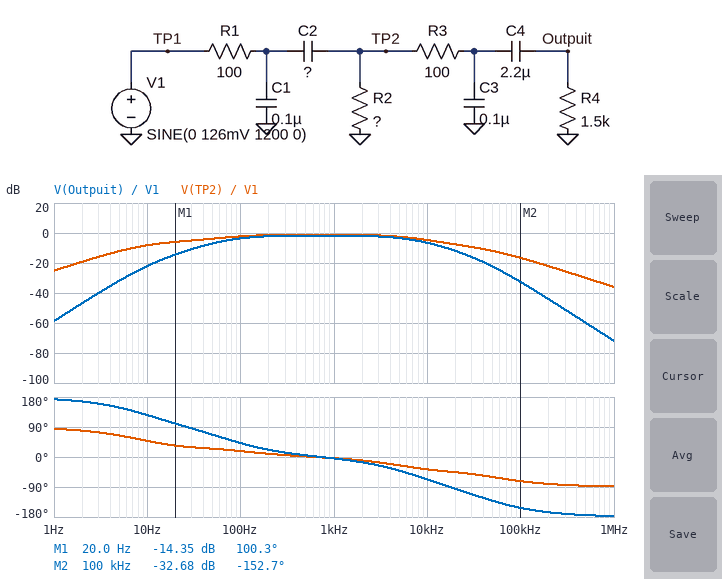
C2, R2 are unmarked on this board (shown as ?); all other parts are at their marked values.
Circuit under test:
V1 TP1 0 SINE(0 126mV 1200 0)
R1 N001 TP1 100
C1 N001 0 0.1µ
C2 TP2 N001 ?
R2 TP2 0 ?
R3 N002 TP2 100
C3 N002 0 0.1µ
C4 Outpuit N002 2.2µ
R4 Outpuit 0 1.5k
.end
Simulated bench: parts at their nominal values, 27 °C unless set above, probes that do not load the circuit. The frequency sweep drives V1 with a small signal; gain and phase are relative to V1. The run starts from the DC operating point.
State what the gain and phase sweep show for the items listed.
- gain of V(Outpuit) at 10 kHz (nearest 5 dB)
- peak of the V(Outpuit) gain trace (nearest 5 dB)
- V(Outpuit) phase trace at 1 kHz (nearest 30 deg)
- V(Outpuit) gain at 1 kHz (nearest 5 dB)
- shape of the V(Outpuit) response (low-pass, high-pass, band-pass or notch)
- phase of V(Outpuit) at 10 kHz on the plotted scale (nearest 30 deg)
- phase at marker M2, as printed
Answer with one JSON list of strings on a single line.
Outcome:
["-5 dB", "0 dB", "0 deg", "0 dB", "band-pass", "-60 deg", "-152.7 deg"]
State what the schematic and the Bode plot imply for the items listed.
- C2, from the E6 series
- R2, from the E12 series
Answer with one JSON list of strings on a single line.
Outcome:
["3.3 µF", "2.7 kΩ"]
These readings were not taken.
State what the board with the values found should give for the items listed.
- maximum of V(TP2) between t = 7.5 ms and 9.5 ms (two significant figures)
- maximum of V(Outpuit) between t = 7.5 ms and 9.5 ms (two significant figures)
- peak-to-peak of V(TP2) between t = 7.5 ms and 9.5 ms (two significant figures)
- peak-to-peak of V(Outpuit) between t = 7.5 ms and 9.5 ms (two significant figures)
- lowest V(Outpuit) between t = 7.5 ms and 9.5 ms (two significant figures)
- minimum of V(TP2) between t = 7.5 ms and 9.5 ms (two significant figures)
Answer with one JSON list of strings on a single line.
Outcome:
["110 mV", "100 mV", "220 mV", "210 mV", "-100 mV", "-110 mV"]
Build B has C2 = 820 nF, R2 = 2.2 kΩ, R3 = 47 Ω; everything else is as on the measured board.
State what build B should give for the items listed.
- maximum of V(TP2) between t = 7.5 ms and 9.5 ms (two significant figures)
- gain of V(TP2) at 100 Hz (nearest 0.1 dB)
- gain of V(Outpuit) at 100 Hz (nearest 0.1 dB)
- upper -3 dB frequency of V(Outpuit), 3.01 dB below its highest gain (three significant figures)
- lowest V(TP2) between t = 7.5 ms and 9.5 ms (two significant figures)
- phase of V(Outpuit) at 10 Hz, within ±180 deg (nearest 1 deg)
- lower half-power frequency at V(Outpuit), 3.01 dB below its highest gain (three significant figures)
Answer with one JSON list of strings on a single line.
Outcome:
["100 mV", "-8.1 dB", "-9.2 dB", "8.64 kHz", "-100 mV", "146 deg", "196 Hz"]
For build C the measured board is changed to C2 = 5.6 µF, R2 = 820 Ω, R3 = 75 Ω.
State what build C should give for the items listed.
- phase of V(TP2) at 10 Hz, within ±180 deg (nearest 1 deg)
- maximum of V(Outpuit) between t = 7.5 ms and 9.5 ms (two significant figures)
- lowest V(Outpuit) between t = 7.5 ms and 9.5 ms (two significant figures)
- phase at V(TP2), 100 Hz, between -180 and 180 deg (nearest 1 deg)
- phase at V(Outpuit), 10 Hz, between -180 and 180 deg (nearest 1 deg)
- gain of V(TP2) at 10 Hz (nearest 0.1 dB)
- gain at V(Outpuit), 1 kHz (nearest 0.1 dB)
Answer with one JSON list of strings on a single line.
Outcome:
["67 deg", "99 mV", "-99 mV", "20 deg", "144 deg", "-11.7 dB", "-2.1 dB"]
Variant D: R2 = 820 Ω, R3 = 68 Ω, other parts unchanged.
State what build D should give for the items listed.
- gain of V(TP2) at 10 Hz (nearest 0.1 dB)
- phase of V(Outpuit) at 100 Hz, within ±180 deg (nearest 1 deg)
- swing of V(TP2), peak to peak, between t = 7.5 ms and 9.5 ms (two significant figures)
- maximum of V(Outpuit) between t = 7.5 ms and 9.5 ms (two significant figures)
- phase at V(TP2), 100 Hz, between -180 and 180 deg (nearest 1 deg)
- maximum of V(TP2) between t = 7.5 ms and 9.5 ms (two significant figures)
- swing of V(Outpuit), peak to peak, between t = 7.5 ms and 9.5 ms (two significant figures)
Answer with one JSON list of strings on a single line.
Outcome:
["-15.9 dB", "56 deg", "210 mV", "98 mV", "31 deg", "100 mV", "200 mV"]
